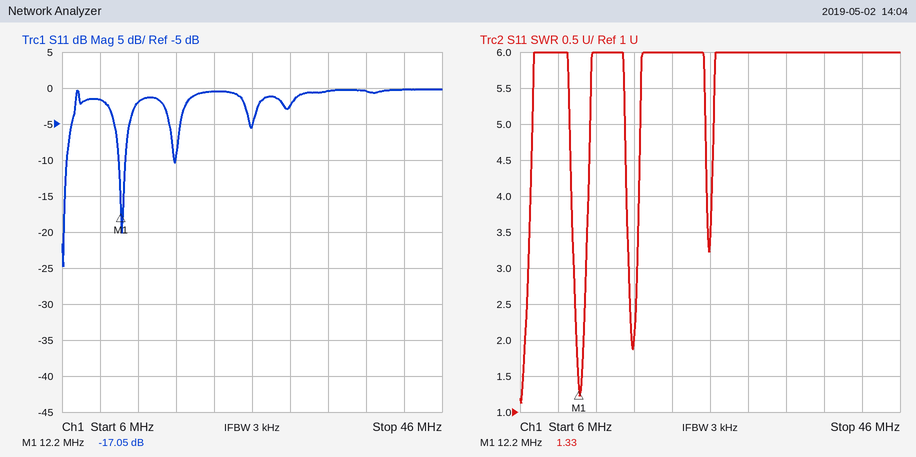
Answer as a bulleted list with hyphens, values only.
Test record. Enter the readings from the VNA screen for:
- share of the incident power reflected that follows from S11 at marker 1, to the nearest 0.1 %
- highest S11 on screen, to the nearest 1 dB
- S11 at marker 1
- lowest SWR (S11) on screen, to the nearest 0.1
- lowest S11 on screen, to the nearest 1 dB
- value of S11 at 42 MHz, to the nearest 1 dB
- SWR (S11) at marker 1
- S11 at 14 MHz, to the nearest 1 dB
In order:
- 2.0 %
- 0 dB
- -17.05 dB
- 1.1
- -25 dB
- 0 dB
- 1.33
- -2 dB
